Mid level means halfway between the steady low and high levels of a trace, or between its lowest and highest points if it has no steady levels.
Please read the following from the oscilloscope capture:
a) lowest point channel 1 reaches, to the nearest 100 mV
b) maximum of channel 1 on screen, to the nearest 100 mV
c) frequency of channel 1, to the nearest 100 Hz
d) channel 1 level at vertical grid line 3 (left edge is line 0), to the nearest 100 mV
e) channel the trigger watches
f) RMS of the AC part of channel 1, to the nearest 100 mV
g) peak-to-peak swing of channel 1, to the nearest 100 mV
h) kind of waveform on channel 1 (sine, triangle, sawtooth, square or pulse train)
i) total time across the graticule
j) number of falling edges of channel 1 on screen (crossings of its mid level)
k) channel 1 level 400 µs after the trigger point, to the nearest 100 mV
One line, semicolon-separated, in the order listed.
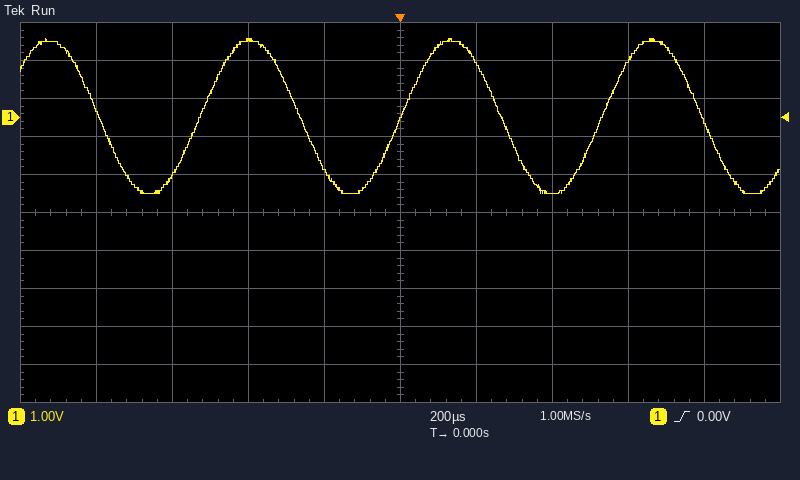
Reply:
-2.0 V; 2.1 V; 1.9 kHz; 2.0 V; channel 1; 1.4 V; 4.1 V; sine; 2 ms; 4; -2.0 V
